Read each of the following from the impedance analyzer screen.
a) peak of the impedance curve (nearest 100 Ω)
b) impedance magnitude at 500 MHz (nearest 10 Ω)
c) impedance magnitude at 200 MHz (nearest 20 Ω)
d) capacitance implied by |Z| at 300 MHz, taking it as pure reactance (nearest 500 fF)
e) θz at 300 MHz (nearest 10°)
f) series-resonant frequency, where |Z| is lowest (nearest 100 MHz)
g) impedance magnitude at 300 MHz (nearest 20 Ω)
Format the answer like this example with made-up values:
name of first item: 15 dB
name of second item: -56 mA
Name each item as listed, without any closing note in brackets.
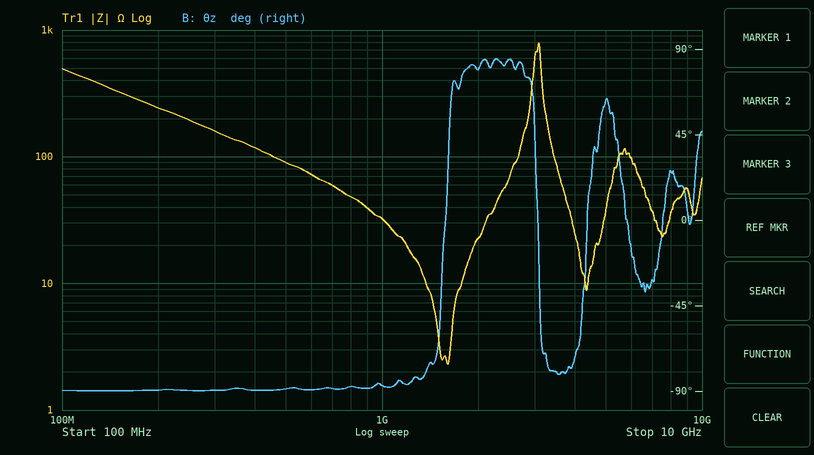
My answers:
peak of the impedance curve: 800 Ω
impedance magnitude at 500 MHz: 90 Ω
impedance magnitude at 200 MHz: 240 Ω
capacitance implied by |Z| at 300 MHz, taking it as pure reactance: 3.5 pF
θz at 300 MHz: -90°
series-resonant frequency, where |Z| is lowest: 1.6 GHz
impedance magnitude at 300 MHz: 160 Ω
